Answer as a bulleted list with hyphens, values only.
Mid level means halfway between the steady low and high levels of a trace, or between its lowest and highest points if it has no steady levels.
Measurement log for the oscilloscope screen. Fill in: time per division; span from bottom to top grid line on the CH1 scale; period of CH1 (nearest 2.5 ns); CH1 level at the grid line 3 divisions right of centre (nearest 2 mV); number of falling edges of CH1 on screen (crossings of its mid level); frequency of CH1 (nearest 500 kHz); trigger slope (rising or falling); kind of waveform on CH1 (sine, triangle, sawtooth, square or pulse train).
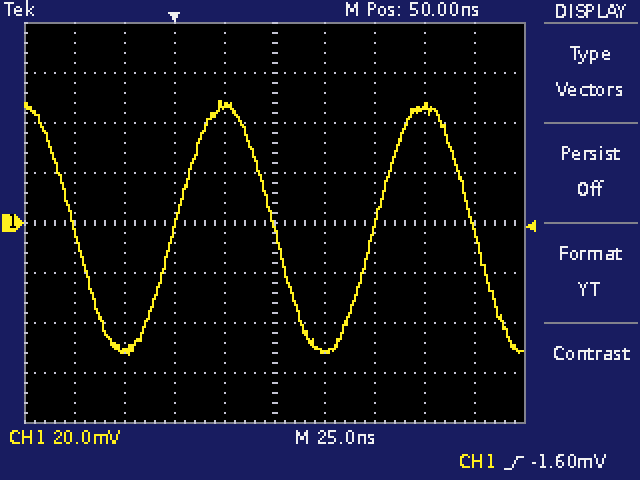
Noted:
- 25 ns
- 160 mV
- 100.0 ns
- 46 mV
- 3
- 10.0 MHz
- rising
- sine
